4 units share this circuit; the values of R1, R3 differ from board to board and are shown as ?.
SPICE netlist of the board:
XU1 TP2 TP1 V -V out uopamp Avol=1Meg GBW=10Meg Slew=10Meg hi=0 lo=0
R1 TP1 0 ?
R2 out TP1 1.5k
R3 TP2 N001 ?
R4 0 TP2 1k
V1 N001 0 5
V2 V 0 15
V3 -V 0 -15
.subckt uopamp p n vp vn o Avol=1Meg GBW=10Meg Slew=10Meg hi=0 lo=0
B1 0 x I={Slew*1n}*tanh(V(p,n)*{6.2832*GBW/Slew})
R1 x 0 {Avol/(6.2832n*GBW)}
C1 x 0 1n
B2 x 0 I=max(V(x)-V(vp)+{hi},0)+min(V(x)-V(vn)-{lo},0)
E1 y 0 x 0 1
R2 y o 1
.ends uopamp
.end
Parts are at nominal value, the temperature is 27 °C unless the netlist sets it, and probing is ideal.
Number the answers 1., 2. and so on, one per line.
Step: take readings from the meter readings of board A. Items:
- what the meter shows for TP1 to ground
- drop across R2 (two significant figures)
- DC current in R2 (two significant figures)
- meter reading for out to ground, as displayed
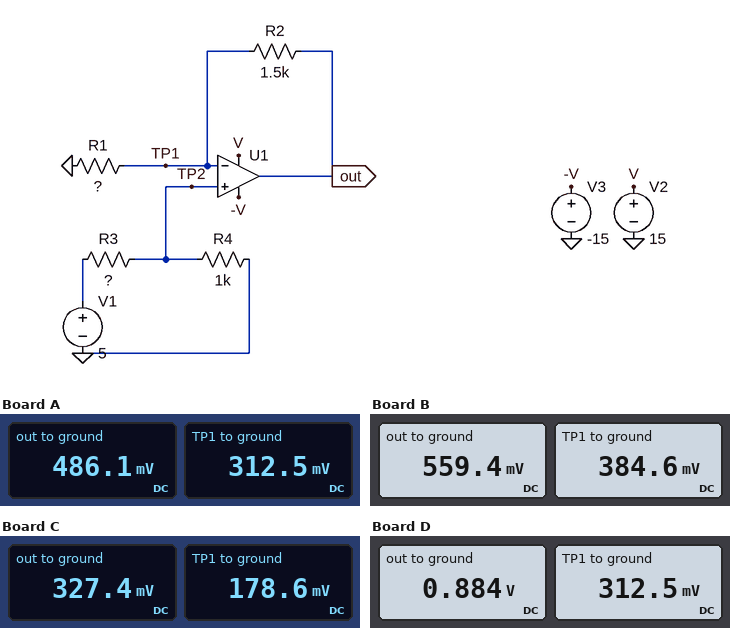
1. 312.5 mV
2. 170 mV
3. 120 µA
4. 486.1 mV
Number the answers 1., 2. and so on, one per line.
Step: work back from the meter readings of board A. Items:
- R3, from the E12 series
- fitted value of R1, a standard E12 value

1. 15 kΩ
2. 2.7 kΩ
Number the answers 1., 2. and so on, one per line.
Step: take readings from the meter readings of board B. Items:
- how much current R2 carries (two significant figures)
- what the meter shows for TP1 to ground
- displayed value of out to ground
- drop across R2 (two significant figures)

1. 120 µA
2. 384.6 mV
3. 559.4 mV
4. 170 mV
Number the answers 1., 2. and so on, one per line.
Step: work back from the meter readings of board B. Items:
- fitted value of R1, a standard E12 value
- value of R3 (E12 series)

1. 3.3 kΩ
2. 12 kΩ
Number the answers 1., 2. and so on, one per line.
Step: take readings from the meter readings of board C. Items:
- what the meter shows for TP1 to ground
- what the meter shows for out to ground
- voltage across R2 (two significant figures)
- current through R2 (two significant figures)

1. 178.6 mV
2. 327.4 mV
3. 150 mV
4. 99 µA
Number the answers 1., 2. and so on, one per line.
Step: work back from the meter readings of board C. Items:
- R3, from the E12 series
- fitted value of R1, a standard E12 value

1. 27 kΩ
2. 1.8 kΩ
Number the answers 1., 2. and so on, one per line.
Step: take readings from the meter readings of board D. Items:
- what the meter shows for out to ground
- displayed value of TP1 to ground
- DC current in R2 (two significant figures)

1. 0.884 V
2. 312.5 mV
3. 380 µA
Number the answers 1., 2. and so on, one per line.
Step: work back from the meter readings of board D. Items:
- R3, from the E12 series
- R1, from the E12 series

1. 15 kΩ
2. 820 Ω
